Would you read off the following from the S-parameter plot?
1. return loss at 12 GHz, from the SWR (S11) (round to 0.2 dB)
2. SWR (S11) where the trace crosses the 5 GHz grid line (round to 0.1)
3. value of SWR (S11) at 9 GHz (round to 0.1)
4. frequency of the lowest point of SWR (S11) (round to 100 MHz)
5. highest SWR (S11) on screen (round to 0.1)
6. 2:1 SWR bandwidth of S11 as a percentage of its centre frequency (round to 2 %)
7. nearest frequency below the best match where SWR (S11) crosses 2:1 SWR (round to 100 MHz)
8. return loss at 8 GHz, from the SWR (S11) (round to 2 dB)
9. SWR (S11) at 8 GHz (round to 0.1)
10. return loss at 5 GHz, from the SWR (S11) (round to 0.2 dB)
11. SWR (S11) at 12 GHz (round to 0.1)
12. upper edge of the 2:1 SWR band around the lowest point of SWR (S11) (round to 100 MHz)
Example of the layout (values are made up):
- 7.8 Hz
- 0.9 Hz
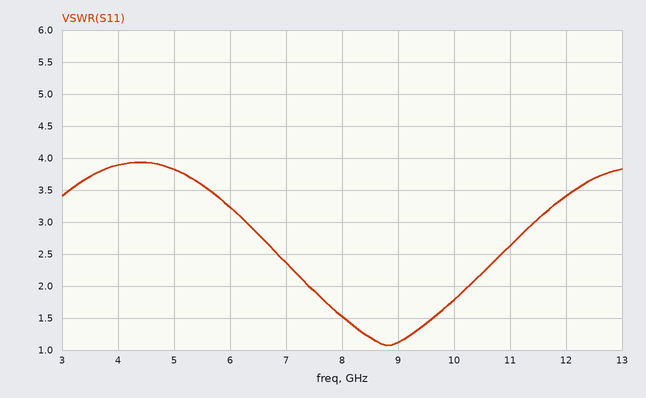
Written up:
- 5.2 dB
- 3.8
- 1.1
- 8.8 GHz
- 3.9
- 32 %
- 7.4 GHz
- 14 dB
- 1.5
- 4.6 dB
- 3.4
- 10.3 GHz
